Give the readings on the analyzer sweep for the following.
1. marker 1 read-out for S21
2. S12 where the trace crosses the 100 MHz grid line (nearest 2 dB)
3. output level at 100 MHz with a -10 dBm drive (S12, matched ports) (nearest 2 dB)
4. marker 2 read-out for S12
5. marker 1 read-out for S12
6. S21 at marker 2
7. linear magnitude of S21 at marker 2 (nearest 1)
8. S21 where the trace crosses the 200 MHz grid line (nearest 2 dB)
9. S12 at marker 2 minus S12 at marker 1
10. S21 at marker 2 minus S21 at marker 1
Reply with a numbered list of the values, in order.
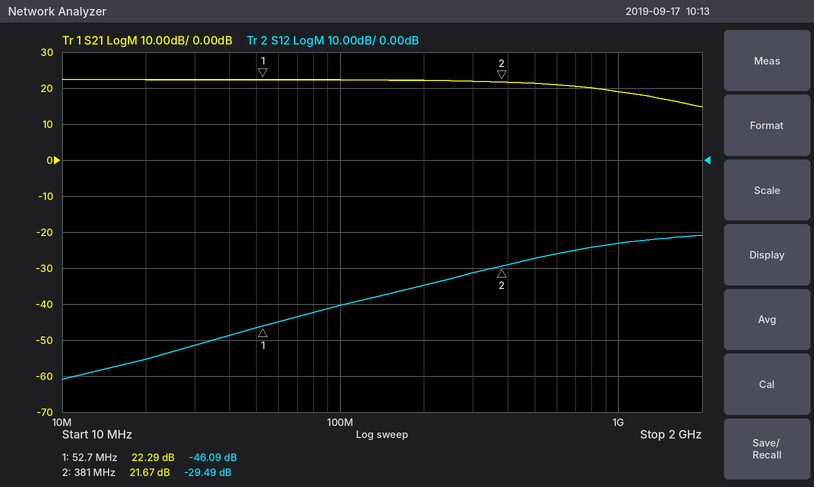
1. 22.29 dB
2. -40 dB
3. -50 dBm
4. -29.49 dB
5. -46.09 dB
6. 21.67 dB
7. 12
8. 22 dB
9. 16.60 dB
10. -0.62 dB
